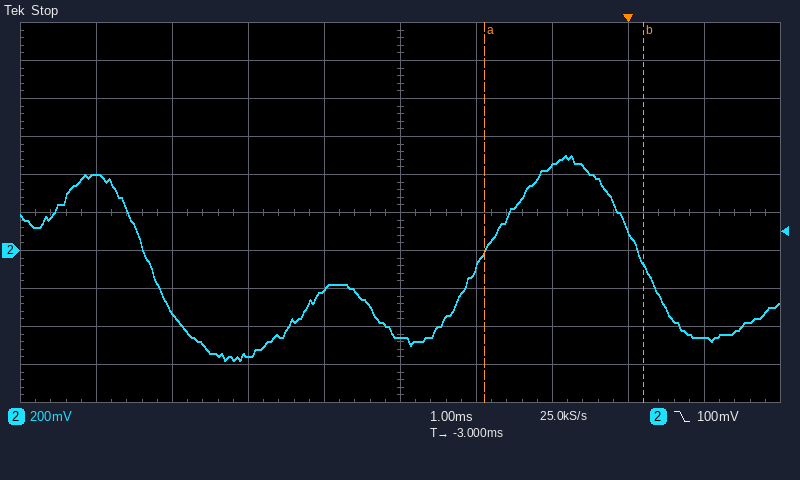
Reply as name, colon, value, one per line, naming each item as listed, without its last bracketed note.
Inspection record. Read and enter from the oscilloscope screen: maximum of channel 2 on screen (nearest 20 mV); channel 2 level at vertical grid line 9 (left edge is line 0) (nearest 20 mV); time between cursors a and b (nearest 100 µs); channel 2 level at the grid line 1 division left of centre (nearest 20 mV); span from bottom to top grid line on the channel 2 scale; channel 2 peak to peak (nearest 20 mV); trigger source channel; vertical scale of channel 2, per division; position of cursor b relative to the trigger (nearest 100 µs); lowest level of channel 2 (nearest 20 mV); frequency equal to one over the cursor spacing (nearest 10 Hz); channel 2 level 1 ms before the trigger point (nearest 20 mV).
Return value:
maximum of channel 2 on screen: 500 mV
channel 2 level at vertical grid line 9 (left edge is line 0): -460 mV
time between cursors a and b: 2.1 ms
channel 2 level at the grid line 1 division left of centre: -200 mV
span from bottom to top grid line on the channel 2 scale: 2 V
channel 2 peak to peak: 1.08 V
trigger source channel: channel 2
vertical scale of channel 2, per division: 200 mV
position of cursor b relative to the trigger: +200 µs
lowest level of channel 2: -580 mV
frequency equal to one over the cursor spacing: 480 Hz
channel 2 level 1 ms before the trigger point: 440 mV
